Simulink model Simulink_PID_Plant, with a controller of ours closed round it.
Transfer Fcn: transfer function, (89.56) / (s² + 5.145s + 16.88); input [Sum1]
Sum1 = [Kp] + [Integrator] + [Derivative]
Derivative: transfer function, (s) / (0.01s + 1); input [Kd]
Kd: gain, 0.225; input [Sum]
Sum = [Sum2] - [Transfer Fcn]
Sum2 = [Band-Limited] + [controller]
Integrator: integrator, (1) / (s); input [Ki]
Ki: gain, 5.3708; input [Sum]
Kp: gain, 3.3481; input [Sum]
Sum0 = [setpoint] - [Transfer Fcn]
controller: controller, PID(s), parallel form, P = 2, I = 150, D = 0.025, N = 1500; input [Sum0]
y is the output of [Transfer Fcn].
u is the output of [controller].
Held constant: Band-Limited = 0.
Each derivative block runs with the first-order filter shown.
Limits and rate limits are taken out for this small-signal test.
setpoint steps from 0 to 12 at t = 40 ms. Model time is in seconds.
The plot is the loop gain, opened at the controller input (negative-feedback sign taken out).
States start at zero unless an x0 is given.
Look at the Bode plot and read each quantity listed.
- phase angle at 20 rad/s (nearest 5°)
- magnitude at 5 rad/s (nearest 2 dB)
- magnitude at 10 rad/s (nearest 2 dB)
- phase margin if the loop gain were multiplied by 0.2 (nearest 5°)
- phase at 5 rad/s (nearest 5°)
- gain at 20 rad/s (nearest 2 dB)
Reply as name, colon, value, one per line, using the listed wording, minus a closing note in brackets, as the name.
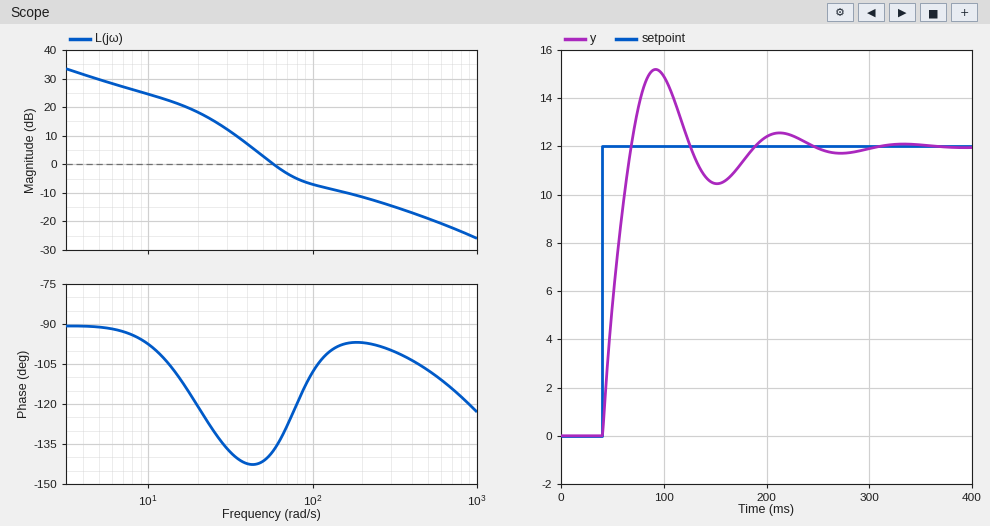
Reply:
phase angle at 20 rad/s: -120°
magnitude at 5 rad/s: 30 dB
magnitude at 10 rad/s: 24 dB
phase margin if the loop gain were multiplied by 0.2: 45°
phase at 5 rad/s: -90°
gain at 20 rad/s: 18 dB
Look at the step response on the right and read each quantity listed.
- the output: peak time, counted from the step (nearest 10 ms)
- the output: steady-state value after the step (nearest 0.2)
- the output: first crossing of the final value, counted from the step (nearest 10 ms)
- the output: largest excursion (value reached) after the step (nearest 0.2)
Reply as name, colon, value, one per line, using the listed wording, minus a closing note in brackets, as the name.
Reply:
the output: peak time, counted from the step: 50 ms
the output: steady-state value after the step: 12.0
the output: first crossing of the final value, counted from the step: 30 ms
the output: largest excursion (value reached) after the step: 15.2
